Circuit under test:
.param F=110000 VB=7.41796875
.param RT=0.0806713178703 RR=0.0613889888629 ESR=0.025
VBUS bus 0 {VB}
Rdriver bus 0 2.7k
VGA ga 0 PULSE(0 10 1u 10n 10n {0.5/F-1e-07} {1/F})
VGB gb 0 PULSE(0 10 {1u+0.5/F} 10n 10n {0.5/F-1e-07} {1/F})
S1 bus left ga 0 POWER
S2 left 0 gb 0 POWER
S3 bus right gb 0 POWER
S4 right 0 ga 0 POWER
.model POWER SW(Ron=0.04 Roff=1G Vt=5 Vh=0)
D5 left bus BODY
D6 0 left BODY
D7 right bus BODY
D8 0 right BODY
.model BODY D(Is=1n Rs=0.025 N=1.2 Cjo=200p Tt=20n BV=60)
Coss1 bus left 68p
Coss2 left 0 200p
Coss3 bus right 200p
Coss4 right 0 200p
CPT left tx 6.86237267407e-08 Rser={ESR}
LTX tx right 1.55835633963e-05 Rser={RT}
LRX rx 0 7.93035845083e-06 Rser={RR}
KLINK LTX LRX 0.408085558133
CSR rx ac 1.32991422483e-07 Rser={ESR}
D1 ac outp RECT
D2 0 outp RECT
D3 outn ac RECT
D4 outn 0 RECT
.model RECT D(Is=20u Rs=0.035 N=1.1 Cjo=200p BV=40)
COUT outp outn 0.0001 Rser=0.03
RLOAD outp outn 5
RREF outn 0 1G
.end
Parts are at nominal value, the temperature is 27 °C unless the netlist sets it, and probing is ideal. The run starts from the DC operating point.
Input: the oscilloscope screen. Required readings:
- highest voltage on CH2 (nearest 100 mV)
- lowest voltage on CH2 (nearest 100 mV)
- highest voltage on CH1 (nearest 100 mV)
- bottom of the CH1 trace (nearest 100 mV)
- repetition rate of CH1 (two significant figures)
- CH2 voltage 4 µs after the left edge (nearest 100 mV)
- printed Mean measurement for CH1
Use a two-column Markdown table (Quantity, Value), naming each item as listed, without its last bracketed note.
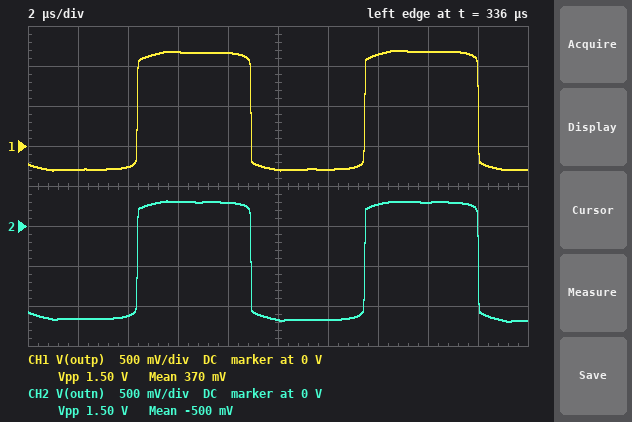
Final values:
| Quantity | Value |
|---|---|
| highest voltage on CH2 | 300 mV |
| lowest voltage on CH2 | -1.2 V |
| highest voltage on CH1 | 1.2 V |
| bottom of the CH1 trace | -300 mV |
| repetition rate of CH1 | 110 kHz |
| CH2 voltage 4 µs after the left edge | -1.1 V |
| printed Mean measurement for CH1 | 370 mV |
